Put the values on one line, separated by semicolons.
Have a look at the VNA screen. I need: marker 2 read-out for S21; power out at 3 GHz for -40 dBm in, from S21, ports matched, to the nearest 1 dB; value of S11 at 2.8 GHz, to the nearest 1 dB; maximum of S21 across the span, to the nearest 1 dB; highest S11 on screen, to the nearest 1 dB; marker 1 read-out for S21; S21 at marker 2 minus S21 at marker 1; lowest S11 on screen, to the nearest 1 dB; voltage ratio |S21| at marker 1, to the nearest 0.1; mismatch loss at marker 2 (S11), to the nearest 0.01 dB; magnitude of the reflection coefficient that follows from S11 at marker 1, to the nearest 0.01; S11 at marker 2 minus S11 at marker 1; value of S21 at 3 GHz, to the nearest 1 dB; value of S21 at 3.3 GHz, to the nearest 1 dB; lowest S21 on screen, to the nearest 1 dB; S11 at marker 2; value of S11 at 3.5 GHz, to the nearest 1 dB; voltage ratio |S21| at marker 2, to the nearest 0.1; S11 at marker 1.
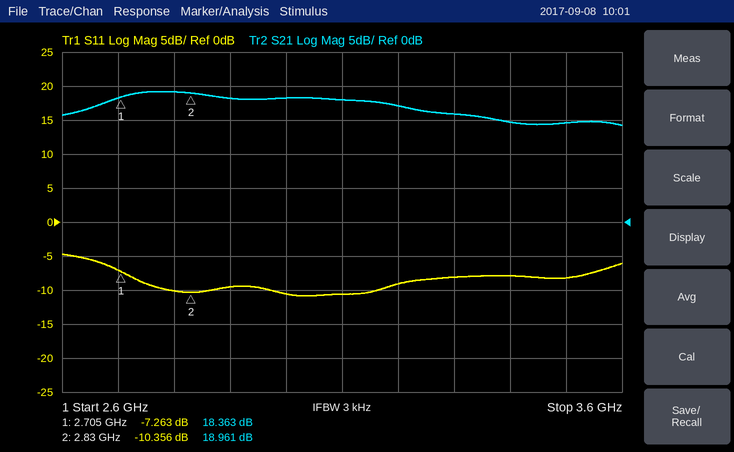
18.961 dB; -22 dBm; -10 dB; 19 dB; -5 dB; 18.363 dB; 0.598 dB; -11 dB; 8.3; 0.42 dB; 0.43; -3.093 dB; 18 dB; 16 dB; 14 dB; -10.356 dB; -8 dB; 8.9; -7.263 dB
